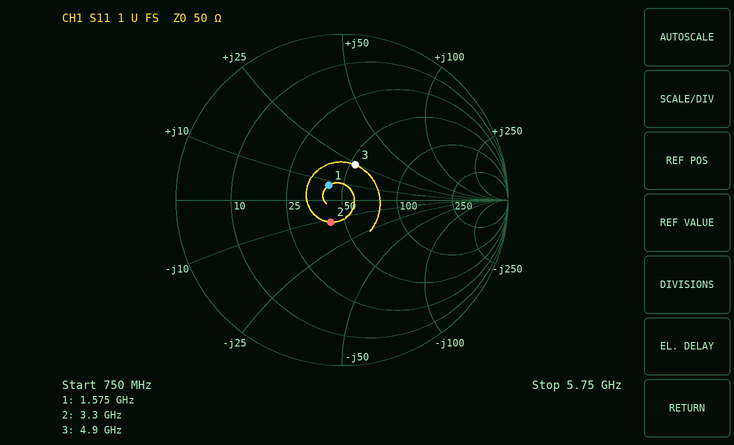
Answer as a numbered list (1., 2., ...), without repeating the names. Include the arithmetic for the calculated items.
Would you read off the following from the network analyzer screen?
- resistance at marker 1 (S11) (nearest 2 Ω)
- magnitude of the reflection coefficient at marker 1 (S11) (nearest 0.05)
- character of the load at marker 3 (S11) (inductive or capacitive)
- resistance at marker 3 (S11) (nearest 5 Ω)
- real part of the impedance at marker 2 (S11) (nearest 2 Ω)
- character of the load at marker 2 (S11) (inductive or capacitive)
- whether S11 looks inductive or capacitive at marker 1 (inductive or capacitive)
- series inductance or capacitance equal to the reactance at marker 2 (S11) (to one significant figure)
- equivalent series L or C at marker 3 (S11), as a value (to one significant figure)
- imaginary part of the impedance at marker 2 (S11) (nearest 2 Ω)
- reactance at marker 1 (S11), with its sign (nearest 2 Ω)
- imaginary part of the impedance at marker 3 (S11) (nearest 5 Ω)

1. 42 Ω
2. 0.10
3. inductive
4. 55 Ω
5. 42 Ω
6. capacitive
7. inductive
8. C = 1/(2π × 3.3 GHz × 12 Ω) ≈ 4 pF
9. L = 25 Ω/(2π × 4.9 GHz) ≈ 812 pH, so 800 pH to one significant figure
10. -12 Ω
11. +8 Ω
12. +25 Ω
